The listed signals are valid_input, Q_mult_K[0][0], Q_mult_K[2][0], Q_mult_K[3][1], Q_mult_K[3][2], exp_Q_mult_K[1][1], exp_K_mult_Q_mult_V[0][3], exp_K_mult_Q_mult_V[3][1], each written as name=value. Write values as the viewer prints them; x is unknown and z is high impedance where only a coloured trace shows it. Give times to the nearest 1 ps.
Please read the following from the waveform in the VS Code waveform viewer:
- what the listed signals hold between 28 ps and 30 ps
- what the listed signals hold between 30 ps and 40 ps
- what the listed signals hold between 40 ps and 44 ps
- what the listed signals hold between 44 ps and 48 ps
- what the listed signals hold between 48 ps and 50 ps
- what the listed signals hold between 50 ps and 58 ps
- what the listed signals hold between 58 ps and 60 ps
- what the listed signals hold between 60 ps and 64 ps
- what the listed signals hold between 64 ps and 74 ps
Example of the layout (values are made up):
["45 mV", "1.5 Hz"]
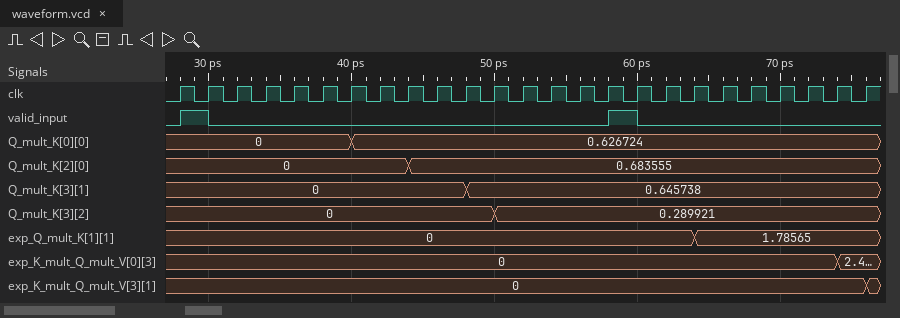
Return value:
["valid_input=1, Q_mult_K[0][0]=0, Q_mult_K[2][0]=0, Q_mult_K[3][1]=0, Q_mult_K[3][2]=0, exp_Q_mult_K[1][1]=0, exp_K_mult_Q_mult_V[0][3]=0, exp_K_mult_Q_mult_V[3][1]=0", "valid_input=0, Q_mult_K[0][0]=0, Q_mult_K[2][0]=0, Q_mult_K[3][1]=0, Q_mult_K[3][2]=0, exp_Q_mult_K[1][1]=0, exp_K_mult_Q_mult_V[0][3]=0, exp_K_mult_Q_mult_V[3][1]=0", "valid_input=0, Q_mult_K[0][0]=0.626724, Q_mult_K[2][0]=0, Q_mult_K[3][1]=0, Q_mult_K[3][2]=0, exp_Q_mult_K[1][1]=0, exp_K_mult_Q_mult_V[0][3]=0, exp_K_mult_Q_mult_V[3][1]=0", "valid_input=0, Q_mult_K[0][0]=0.626724, Q_mult_K[2][0]=0.683555, Q_mult_K[3][1]=0, Q_mult_K[3][2]=0, exp_Q_mult_K[1][1]=0, exp_K_mult_Q_mult_V[0][3]=0, exp_K_mult_Q_mult_V[3][1]=0", "valid_input=0, Q_mult_K[0][0]=0.626724, Q_mult_K[2][0]=0.683555, Q_mult_K[3][1]=0.645738, Q_mult_K[3][2]=0, exp_Q_mult_K[1][1]=0, exp_K_mult_Q_mult_V[0][3]=0, exp_K_mult_Q_mult_V[3][1]=0", "valid_input=0, Q_mult_K[0][0]=0.626724, Q_mult_K[2][0]=0.683555, Q_mult_K[3][1]=0.645738, Q_mult_K[3][2]=0.289921, exp_Q_mult_K[1][1]=0, exp_K_mult_Q_mult_V[0][3]=0, exp_K_mult_Q_mult_V[3][1]=0", "valid_input=1, Q_mult_K[0][0]=0.626724, Q_mult_K[2][0]=0.683555, Q_mult_K[3][1]=0.645738, Q_mult_K[3][2]=0.289921, exp_Q_mult_K[1][1]=0, exp_K_mult_Q_mult_V[0][3]=0, exp_K_mult_Q_mult_V[3][1]=0", "valid_input=0, Q_mult_K[0][0]=0.626724, Q_mult_K[2][0]=0.683555, Q_mult_K[3][1]=0.645738, Q_mult_K[3][2]=0.289921, exp_Q_mult_K[1][1]=0, exp_K_mult_Q_mult_V[0][3]=0, exp_K_mult_Q_mult_V[3][1]=0", "valid_input=0, Q_mult_K[0][0]=0.626724, Q_mult_K[2][0]=0.683555, Q_mult_K[3][1]=0.645738, Q_mult_K[3][2]=0.289921, exp_Q_mult_K[1][1]=1.78565, exp_K_mult_Q_mult_V[0][3]=0, exp_K_mult_Q_mult_V[3][1]=0"]
